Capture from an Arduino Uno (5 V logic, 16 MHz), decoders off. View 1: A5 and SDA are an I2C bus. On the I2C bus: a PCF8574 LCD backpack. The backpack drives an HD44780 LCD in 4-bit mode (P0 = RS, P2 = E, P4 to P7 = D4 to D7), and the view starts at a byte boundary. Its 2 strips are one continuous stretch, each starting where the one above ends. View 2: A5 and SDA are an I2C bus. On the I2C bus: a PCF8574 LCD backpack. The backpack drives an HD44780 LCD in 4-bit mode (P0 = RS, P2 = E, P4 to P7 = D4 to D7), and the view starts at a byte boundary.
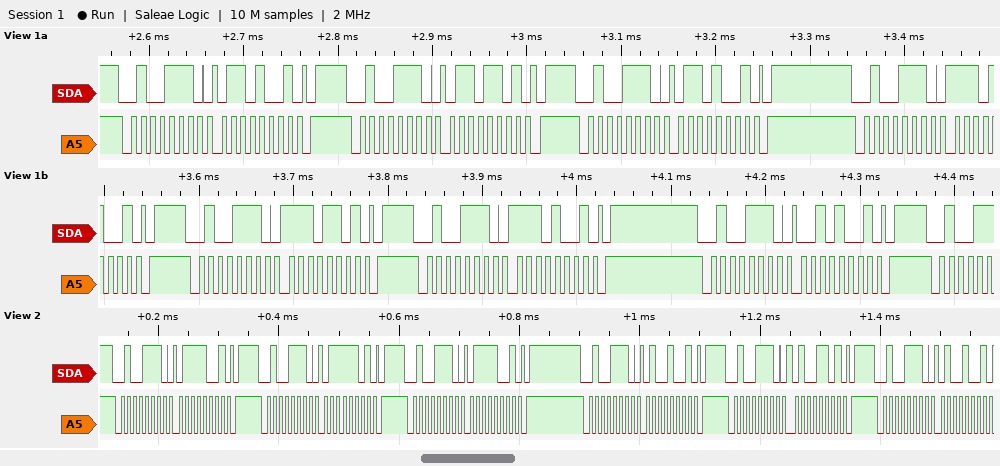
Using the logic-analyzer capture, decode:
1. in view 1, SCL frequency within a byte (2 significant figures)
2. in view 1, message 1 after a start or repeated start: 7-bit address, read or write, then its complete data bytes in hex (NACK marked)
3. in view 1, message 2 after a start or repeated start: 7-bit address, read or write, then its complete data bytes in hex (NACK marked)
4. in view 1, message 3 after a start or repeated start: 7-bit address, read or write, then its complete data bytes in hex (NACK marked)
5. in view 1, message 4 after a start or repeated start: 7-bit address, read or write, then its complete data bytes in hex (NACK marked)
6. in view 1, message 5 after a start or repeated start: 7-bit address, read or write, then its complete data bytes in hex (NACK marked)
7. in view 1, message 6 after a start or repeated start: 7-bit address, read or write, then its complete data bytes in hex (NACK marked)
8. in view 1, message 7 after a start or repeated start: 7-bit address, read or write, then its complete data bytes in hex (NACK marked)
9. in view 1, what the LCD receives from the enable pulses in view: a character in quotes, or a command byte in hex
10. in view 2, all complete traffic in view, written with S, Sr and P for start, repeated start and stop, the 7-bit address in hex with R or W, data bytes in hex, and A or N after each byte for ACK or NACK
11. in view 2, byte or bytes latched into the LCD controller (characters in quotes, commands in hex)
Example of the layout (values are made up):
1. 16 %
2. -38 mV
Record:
1. 100 kHz
2. 0x27 write: 69
3. 0x27 write: 6D
4. 0x27 write: 69
5. 0x27 write: E9
6. 0x27 write: ED
7. 0x27 write: E9
8. 0x27 write: 29
9. 'n'
10. S 27W A 79 A P S 27W A 7D A P S 27W A 79 A P S 27W A 49 A P S 27W A 4D A P S 27W A 49 A
11. 't'
